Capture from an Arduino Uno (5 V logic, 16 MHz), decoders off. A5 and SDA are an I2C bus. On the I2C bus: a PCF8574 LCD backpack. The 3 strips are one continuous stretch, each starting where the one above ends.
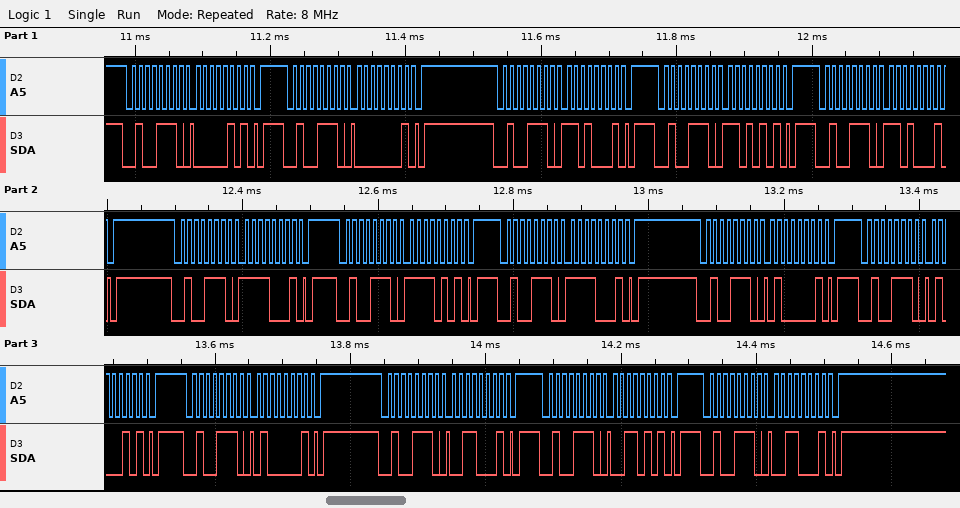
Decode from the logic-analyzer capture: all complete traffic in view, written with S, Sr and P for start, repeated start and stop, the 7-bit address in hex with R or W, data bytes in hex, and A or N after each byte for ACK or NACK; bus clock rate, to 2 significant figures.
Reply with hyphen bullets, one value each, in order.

- S 27W A 05 A P S 27W A 01 A P S 27W A D1 A P S 27W A D5 A P S 27W A D1 A P S 27W A F1 A P S 27W A F5 A P S 27W A F1 A P S 27W A 41 A P S 27W A 45 A P S 27W A 41 A P S 27W A 31 A P S 27W A 35 A P S 27W A 31 A P
- 100 kHz
